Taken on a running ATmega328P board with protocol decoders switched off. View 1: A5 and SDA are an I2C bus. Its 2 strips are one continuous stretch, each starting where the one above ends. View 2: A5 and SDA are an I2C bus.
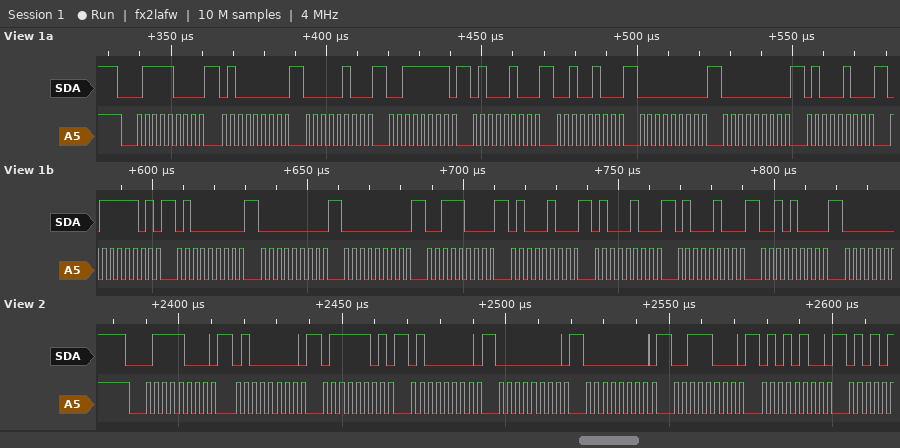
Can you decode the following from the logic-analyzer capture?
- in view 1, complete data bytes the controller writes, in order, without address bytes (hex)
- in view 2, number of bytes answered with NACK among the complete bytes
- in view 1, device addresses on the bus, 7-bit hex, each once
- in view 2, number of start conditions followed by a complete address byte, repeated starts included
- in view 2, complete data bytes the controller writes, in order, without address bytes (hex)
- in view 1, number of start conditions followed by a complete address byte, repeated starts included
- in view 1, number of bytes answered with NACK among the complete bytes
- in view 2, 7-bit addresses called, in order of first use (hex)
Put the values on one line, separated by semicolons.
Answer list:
40 04 3F 44 24 00 00 44 7D 40 00 00 38 44 44 44 28; 0; 0x3C; 1; 40 7D 40 00 00 38 54; 1; 0; 0x3C
